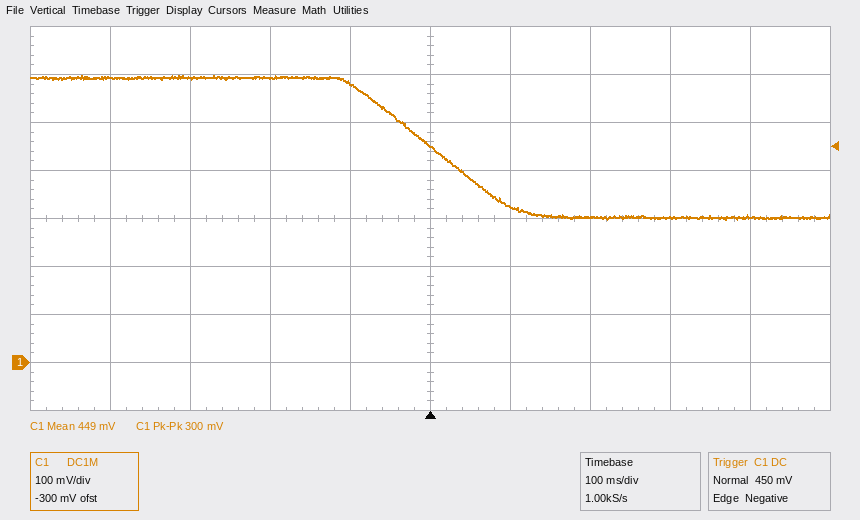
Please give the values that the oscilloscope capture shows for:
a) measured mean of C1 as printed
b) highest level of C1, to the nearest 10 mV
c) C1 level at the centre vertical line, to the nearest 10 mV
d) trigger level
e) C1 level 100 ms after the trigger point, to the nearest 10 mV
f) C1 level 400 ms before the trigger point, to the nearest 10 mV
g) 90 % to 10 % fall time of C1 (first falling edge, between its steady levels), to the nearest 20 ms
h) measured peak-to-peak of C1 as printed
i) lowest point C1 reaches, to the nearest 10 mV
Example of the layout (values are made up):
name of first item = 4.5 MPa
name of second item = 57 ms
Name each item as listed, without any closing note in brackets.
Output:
measured mean of C1 as printed = 449 mV
highest level of C1, to the nearest 10 mV = 600 mV
C1 level at the centre vertical line, to the nearest 10 mV = 450 mV
trigger level = 450 mV
C1 level 100 ms after the trigger point, to the nearest 10 mV = 320 mV
C1 level 400 ms before the trigger point, to the nearest 10 mV = 590 mV
90 % to 10 % fall time of C1 (first falling edge, between its steady levels), to the nearest 20 ms = 180 ms
measured peak-to-peak of C1 as printed = 300 mV
lowest point C1 reaches, to the nearest 10 mV = 300 mV
